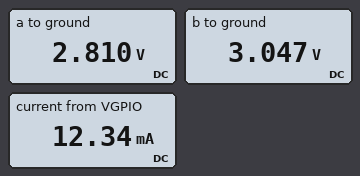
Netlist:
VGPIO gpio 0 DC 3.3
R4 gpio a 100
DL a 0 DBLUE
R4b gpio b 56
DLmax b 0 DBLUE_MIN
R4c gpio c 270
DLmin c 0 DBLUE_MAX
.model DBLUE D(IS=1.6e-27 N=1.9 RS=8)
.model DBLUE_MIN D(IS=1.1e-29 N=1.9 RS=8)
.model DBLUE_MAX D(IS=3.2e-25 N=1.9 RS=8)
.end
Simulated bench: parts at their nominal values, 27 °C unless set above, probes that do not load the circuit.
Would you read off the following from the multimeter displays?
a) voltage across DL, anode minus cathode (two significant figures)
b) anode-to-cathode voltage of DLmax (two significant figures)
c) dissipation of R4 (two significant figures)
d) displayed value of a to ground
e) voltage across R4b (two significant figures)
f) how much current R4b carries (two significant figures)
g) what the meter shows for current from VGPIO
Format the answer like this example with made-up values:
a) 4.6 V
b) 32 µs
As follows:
a) 2.8 V
b) 3.0 V
c) 2.4 mW
d) 2.810 V
e) 250 mV
f) 4.5 mA
g) 12.34 mA
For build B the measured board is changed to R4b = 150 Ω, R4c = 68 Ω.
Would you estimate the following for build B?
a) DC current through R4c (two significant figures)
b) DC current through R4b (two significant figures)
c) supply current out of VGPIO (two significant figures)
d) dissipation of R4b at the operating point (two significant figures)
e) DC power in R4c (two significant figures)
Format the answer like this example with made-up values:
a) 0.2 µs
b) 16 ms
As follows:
a) 9.9 mA
b) 2.1 mA
c) 17 mA
d) 640 µW
e) 6.7 mW
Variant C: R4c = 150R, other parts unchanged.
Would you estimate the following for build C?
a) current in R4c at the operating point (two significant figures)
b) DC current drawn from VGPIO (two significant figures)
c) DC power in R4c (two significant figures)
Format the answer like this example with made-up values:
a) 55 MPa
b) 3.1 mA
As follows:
a) 5.0 mA
b) 14 mA
c) 3.7 mW
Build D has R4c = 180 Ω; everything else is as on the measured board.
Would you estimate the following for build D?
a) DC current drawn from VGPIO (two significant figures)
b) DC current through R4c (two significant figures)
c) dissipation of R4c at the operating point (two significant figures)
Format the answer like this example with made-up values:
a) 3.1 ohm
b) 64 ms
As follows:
a) 14 mA
b) 4.2 mA
c) 3.2 mW
